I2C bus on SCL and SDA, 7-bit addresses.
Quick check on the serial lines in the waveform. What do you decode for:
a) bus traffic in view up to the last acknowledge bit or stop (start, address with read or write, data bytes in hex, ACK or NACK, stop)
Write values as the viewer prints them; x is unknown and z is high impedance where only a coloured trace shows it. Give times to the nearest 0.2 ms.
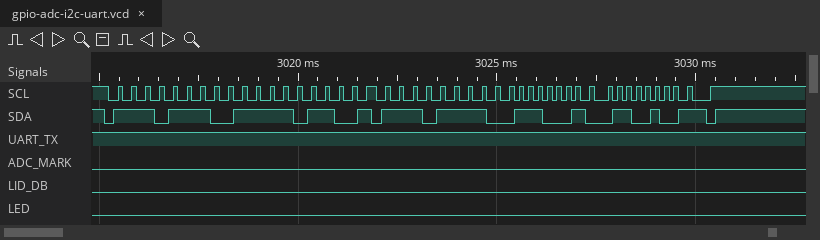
start, address 77 write ACK, F6 ACK, repeated start, address 77 read ACK, 71 ACK, 64 NACK, stop
